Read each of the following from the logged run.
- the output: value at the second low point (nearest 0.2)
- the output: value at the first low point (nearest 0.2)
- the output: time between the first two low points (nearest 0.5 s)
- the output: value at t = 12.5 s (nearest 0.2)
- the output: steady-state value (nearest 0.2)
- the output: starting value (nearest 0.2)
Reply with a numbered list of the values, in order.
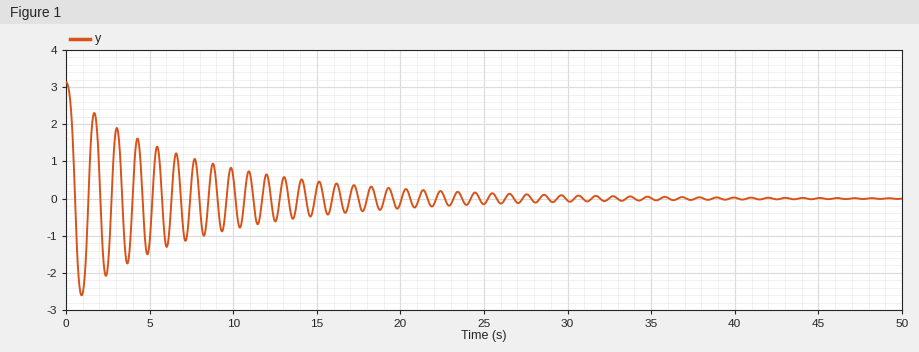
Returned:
1. -2.0
2. -2.6
3. 1.5 s
4. -0.6
5. 0.0
6. 3.2
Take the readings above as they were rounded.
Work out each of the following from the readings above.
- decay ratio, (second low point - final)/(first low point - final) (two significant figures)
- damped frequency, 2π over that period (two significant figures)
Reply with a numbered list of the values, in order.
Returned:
1. 0.77
2. 4.2 rad/s
